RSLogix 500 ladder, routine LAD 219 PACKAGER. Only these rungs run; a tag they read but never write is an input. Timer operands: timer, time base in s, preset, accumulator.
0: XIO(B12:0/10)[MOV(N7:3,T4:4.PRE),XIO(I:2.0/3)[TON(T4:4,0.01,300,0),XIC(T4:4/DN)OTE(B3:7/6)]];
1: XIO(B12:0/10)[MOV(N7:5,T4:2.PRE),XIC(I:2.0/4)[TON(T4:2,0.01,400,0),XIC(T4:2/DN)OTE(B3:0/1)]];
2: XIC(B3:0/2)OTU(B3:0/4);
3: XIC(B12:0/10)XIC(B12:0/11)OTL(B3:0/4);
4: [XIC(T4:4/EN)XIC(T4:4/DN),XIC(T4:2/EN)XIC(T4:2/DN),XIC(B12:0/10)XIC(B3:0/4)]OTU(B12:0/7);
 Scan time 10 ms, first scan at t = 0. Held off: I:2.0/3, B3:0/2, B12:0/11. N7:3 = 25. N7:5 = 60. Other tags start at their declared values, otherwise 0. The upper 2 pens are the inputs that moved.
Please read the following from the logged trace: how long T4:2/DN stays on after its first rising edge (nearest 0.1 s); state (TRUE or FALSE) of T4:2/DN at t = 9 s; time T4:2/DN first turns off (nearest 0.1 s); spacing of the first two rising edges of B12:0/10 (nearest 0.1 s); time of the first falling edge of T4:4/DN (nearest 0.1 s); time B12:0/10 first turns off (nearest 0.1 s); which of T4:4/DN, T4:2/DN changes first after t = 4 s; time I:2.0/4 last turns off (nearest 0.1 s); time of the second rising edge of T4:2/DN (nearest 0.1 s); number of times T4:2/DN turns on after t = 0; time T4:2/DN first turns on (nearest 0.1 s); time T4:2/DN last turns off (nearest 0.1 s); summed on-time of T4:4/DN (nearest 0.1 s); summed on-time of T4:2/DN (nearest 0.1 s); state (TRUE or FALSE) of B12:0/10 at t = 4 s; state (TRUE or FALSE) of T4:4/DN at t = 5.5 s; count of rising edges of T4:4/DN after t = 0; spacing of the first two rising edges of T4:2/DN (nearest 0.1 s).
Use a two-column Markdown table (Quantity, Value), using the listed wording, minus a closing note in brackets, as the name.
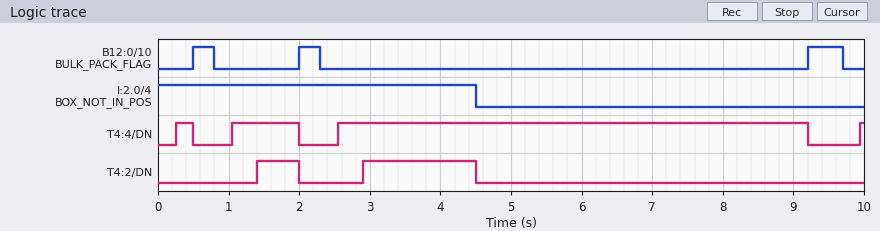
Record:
| Quantity | Value |
|---|---|
| how long T4:2/DN stays on after its first rising edge | 0.6 s |
| state (TRUE or FALSE) of T4:2/DN at t = 9 s | FALSE |
| time T4:2/DN first turns off | 2.0 s |
| spacing of the first two rising edges of B12:0/10 | 1.5 s |
| time of the first falling edge of T4:4/DN | 0.5 s |
| time B12:0/10 first turns off | 0.8 s |
| which of T4:4/DN, T4:2/DN changes first after t = 4 s | T4:2/DN |
| time I:2.0/4 last turns off | 4.5 s |
| time of the second rising edge of T4:2/DN | 2.9 s |
| number of times T4:2/DN turns on after t = 0 | 2 |
| time T4:2/DN first turns on | 1.4 s |
| time T4:2/DN last turns off | 4.5 s |
| summed on-time of T4:4/DN | 7.9 s |
| summed on-time of T4:2/DN | 2.2 s |
| state (TRUE or FALSE) of B12:0/10 at t = 4 s | FALSE |
| state (TRUE or FALSE) of T4:4/DN at t = 5.5 s | TRUE |
| count of rising edges of T4:4/DN after t = 0 | 4 |
| spacing of the first two rising edges of T4:2/DN | 1.5 s |
